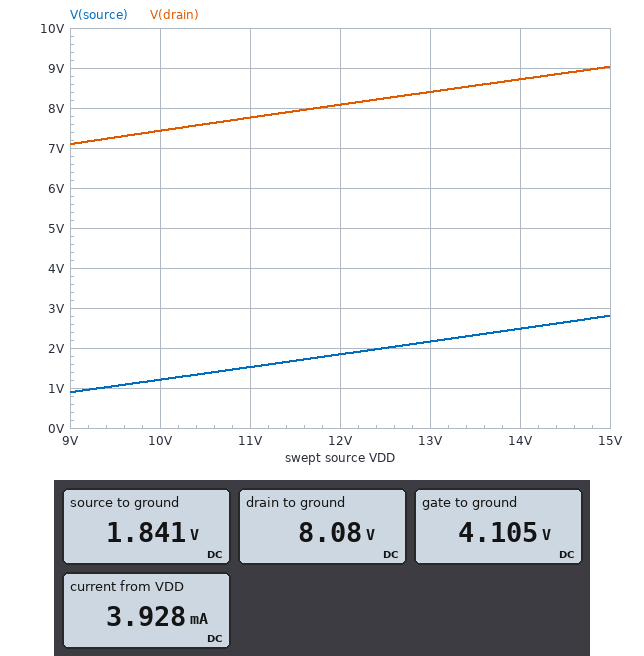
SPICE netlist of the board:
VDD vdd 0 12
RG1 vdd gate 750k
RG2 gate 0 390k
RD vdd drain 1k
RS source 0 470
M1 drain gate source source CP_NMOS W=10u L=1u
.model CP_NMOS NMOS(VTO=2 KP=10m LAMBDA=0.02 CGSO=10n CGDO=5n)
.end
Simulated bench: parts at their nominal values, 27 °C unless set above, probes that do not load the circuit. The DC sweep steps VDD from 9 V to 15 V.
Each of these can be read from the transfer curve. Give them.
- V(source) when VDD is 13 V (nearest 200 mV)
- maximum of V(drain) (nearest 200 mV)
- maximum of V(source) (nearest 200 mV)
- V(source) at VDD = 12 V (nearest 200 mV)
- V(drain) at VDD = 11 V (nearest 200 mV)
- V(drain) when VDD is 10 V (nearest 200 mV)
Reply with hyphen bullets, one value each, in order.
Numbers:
- 2.2 V
- 9.0 V
- 2.8 V
- 1.8 V
- 7.8 V
- 7.4 V
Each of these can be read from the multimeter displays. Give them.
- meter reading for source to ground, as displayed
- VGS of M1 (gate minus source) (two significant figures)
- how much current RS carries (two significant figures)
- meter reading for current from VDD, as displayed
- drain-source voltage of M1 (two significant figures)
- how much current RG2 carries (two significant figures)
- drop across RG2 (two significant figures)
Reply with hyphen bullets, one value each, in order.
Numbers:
- 1.841 V
- 2.3 V
- 3.9 mA
- 3.928 mA
- 6.2 V
- 11 µA
- 4.1 V
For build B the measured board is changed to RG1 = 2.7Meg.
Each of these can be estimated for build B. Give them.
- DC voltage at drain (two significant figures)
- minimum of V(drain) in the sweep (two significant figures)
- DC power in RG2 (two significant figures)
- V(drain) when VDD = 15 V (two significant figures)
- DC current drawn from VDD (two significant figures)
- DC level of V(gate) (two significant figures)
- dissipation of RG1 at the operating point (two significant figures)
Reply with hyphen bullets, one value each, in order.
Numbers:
- 12 V
- 9.0 V
- 5.9 µW
- 15 V
- 3.9 µA
- 1.5 V
- 41 µW
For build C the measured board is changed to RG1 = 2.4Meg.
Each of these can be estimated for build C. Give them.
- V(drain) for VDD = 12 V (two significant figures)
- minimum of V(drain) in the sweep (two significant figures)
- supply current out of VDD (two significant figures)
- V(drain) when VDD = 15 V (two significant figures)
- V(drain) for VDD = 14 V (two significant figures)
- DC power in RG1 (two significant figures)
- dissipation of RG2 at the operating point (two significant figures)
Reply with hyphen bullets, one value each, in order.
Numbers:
- 12 V
- 9.0 V
- 4.3 µA
- 15 V
- 14 V
- 44 µW
- 7.2 µW
